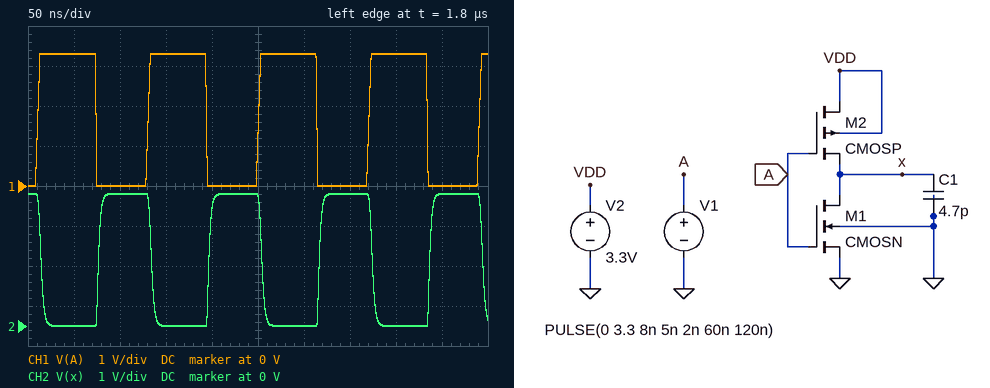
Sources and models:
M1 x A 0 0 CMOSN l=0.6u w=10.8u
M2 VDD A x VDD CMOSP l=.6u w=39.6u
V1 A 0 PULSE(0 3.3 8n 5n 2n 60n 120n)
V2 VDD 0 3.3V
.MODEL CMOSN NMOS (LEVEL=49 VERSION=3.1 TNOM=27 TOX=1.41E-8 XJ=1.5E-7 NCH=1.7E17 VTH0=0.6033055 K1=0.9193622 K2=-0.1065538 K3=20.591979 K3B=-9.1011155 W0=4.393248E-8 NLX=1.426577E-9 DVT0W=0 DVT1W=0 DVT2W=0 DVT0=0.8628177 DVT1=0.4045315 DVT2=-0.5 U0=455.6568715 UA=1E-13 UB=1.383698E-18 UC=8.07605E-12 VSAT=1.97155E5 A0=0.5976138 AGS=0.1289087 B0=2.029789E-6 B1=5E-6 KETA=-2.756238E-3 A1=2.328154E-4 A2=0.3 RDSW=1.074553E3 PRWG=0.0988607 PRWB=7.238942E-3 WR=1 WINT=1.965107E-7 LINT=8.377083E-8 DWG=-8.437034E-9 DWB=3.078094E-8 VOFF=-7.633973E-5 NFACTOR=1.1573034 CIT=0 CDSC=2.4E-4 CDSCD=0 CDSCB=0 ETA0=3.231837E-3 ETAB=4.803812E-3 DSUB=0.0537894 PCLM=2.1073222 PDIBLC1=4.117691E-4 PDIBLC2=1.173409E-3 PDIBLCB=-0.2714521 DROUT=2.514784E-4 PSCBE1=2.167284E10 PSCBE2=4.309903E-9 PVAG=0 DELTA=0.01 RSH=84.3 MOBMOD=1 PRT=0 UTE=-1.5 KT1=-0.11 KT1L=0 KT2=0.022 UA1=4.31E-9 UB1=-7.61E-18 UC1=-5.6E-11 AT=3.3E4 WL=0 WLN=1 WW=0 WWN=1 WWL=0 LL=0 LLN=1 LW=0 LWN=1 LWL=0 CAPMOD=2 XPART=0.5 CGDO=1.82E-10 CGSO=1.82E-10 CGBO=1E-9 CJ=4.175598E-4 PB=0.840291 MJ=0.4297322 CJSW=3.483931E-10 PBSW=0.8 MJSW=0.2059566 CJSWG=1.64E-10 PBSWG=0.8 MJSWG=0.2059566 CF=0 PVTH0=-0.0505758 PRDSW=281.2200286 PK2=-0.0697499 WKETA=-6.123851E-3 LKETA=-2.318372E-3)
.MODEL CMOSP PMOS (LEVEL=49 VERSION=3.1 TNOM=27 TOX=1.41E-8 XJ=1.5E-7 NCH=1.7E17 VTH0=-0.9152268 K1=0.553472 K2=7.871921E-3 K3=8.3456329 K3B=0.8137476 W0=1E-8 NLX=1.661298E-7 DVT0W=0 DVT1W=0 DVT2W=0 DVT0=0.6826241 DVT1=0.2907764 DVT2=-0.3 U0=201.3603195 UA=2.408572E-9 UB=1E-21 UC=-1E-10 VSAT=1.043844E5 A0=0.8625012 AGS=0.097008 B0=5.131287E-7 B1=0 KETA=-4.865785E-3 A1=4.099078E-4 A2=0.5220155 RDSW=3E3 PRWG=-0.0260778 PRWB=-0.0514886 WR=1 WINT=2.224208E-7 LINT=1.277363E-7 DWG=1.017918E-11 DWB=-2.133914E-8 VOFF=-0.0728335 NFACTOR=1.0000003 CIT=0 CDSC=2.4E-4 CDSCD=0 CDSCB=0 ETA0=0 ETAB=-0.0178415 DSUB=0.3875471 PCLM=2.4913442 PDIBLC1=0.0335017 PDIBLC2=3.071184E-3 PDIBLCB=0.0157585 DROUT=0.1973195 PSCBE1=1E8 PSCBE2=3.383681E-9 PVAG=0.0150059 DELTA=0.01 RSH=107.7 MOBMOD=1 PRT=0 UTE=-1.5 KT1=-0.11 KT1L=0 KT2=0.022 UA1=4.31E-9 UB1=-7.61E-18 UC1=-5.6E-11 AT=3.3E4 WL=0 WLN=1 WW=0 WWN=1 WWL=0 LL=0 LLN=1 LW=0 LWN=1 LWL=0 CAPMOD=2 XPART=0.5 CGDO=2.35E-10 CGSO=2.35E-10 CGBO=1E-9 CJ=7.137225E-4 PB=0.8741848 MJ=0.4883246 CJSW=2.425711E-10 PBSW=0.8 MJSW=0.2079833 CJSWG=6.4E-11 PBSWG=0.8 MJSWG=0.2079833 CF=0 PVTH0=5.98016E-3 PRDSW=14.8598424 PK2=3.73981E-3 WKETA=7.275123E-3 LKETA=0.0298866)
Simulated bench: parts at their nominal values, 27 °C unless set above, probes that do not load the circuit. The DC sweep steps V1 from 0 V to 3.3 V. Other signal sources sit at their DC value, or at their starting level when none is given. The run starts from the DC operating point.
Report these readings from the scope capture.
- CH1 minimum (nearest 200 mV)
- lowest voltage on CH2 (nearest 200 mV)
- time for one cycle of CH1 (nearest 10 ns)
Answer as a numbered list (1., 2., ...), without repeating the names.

1. 0 V
2. 0 V
3. 120 ns
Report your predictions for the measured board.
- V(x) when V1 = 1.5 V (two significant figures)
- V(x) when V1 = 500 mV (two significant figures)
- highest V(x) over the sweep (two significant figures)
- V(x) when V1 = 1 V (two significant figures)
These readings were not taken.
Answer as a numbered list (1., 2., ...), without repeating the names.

1. 2.7 V
2. 3.3 V
3. 3.3 V
4. 3.2 V
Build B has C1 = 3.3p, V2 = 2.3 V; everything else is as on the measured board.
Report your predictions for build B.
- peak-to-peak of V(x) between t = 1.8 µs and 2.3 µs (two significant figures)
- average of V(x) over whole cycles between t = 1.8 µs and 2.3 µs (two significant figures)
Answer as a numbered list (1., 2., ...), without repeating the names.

1. 2.3 V
2. 1.1 V
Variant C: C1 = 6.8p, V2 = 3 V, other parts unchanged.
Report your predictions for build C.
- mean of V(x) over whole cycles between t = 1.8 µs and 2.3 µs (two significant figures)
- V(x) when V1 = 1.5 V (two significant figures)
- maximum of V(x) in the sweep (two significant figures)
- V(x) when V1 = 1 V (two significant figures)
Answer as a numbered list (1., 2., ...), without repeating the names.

1. 1.4 V
2. 600 mV
3. 3.0 V
4. 2.9 V
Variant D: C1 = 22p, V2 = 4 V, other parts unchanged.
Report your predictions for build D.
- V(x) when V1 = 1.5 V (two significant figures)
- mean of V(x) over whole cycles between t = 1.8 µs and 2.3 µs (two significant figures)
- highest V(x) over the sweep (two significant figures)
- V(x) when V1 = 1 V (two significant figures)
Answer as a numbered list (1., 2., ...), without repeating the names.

1. 3.6 V
2. 2.1 V
3. 4.0 V
4. 3.9 V
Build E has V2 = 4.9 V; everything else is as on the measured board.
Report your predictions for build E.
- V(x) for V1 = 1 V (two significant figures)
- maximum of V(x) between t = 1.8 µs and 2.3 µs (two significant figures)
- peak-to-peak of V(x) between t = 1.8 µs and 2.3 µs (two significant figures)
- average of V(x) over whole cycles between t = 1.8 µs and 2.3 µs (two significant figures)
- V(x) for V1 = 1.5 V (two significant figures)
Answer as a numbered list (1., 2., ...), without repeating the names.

1. 4.8 V
2. 4.9 V
3. 4.5 V
4. 2.7 V
5. 4.6 V
